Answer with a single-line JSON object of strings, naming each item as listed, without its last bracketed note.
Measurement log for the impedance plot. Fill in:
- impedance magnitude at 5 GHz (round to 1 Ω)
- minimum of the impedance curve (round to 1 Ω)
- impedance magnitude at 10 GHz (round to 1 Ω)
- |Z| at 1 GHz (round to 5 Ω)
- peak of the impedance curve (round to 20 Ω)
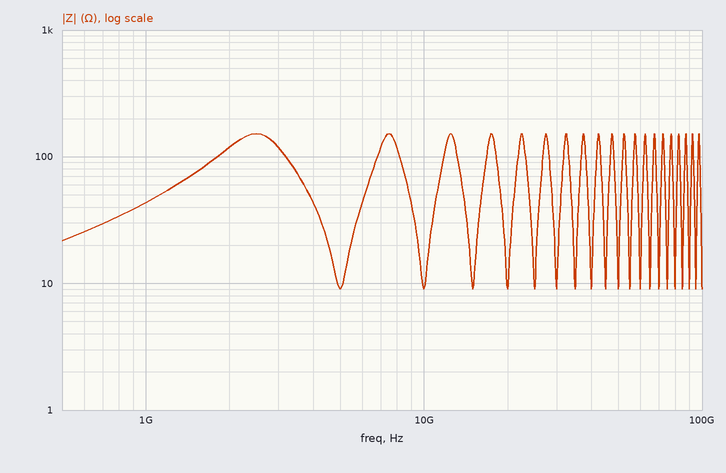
{"impedance magnitude at 5 GHz": "9 Ω", "minimum of the impedance curve": "9 Ω", "impedance magnitude at 10 GHz": "9 Ω", "|Z| at 1 GHz": "45 Ω", "peak of the impedance curve": "160 Ω"}
